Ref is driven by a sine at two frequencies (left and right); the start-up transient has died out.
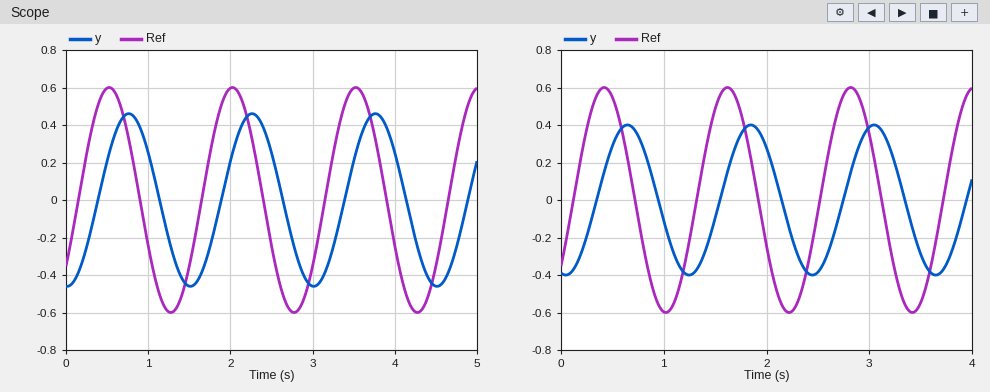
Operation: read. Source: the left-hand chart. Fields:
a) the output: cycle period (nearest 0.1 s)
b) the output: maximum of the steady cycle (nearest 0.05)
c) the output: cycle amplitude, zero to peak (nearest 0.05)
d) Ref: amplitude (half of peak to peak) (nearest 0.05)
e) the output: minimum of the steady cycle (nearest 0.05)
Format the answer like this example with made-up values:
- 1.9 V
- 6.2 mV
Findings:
- 1.5 s
- 0.45
- 0.45
- 0.60
- -0.45
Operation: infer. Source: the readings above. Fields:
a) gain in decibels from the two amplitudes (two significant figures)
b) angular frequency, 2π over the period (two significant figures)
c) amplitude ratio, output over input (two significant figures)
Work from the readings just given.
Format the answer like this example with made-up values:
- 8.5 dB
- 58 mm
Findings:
- -2.5 dB
- 4.2 rad/s
- 0.75
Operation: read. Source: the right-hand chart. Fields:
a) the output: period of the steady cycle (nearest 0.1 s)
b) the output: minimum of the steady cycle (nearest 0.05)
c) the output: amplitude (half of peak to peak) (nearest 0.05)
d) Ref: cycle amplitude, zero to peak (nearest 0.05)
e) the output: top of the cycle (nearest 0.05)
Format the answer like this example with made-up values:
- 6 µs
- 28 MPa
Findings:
- 1.2 s
- -0.40
- 0.40
- 0.60
- 0.40
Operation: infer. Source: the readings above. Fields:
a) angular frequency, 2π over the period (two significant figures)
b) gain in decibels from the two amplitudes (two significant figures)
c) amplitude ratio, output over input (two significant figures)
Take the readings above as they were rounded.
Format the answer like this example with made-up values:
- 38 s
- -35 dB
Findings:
- 5.2 rad/s
- -3.5 dB
- 0.67
